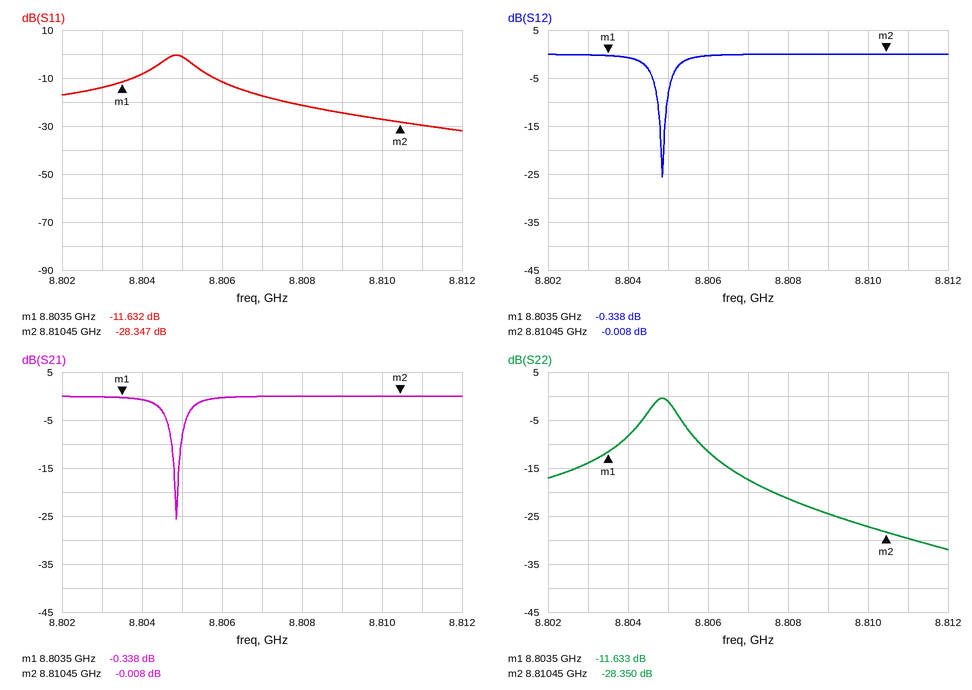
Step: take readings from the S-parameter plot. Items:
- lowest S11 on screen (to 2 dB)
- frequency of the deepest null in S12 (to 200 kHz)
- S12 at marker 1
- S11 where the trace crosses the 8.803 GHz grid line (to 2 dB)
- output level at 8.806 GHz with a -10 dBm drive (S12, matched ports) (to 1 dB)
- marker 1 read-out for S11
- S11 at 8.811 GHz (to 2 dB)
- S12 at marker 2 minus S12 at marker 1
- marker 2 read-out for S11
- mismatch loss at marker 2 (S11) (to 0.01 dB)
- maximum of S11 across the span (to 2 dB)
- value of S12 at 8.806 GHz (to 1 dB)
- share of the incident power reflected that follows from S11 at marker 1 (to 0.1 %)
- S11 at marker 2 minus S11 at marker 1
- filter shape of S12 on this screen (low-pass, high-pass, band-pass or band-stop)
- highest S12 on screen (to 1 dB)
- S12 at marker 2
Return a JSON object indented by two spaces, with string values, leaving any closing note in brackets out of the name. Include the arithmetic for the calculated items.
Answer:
{
  "lowest S11 on screen": "-32 dB",
  "frequency of the deepest null in S12": "8.8048 GHz",
  "S12 at marker 1": "-0.338 dB",
  "S11 where the trace crosses the 8.803 GHz grid line": "-14 dB",
  "output level at 8.806 GHz with a -10 dBm drive (S12, matched ports)": "-10 dBm + (0 dB) = -10 dBm",
  "marker 1 read-out for S11": "-11.632 dB",
  "S11 at 8.811 GHz": "-30 dB",
  "S12 at marker 2 minus S12 at marker 1": "-0.008 − (-0.338) = 0.330 dB",
  "marker 2 read-out for S11": "-28.347 dB",
  "mismatch loss at marker 2 (S11)": "−10 log10(1 − 10^(-28.347/10)) ≈ 0.01 dB",
  "maximum of S11 across the span": "0 dB",
  "value of S12 at 8.806 GHz": "0 dB",
  "share of the incident power reflected that follows from S11 at marker 1": "10^(-11.632/10) ≈ 6.9 %",
  "S11 at marker 2 minus S11 at marker 1": "-28.347 − (-11.632) = -16.715 dB",
  "filter shape of S12 on this screen": "band-stop",
  "highest S12 on screen": "0 dB",
  "S12 at marker 2": "-0.008 dB"
}
